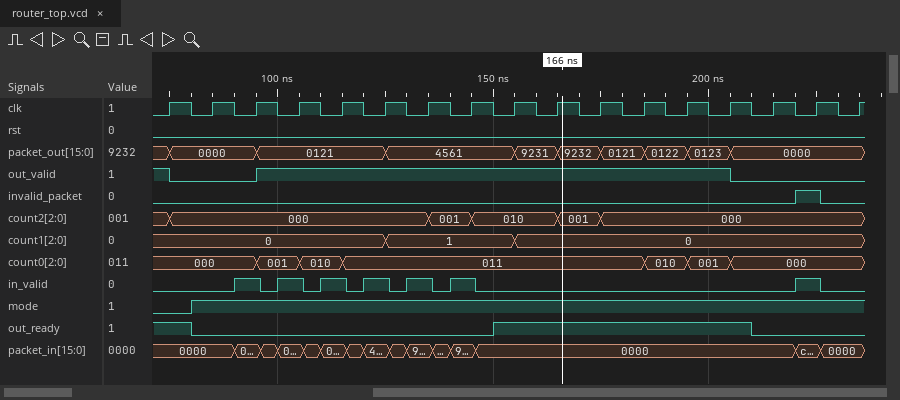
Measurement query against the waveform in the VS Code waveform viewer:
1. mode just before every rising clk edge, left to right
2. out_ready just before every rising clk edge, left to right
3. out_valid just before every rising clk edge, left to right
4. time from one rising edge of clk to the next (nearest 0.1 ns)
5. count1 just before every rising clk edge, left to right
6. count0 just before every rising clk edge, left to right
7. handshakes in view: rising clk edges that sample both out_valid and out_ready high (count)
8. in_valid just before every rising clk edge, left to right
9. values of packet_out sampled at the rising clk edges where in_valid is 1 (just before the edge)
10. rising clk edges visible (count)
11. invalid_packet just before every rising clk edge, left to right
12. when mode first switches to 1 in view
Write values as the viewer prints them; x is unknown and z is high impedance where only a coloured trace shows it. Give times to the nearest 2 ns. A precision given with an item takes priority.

0 1 1 1 1 1 1 1 1 1 1 1 1 1 1 1 1
1 0 0 0 0 0 0 0 1 1 1 1 1 1 0 0 0
1 0 0 1 1 1 1 1 1 1 1 1 1 1 0 0 0
10 ns
0, 0, 0, 0, 0, 0, 1, 1, 1, 0, 0, 0, 0, 0, 0, 0, 0
000, 000, 000, 001, 010, 011, 011, 011, 011, 011, 011, 011, 010, 001, 000, 000, 000
7
0 0 1 1 1 1 1 1 0 0 0 0 0 0 0 1 0
0000, 0121, 0121, 0121, 4561, 4561, 0000
17
0 0 0 0 0 0 0 0 0 0 0 0 0 0 0 1 0
80 ns
